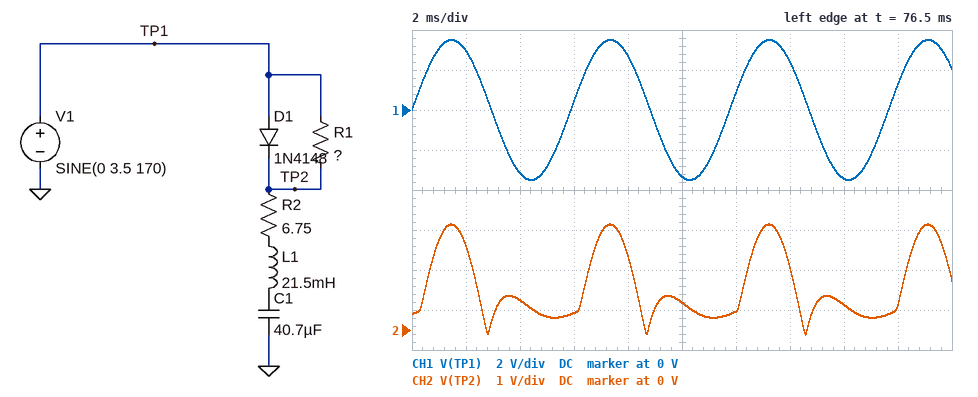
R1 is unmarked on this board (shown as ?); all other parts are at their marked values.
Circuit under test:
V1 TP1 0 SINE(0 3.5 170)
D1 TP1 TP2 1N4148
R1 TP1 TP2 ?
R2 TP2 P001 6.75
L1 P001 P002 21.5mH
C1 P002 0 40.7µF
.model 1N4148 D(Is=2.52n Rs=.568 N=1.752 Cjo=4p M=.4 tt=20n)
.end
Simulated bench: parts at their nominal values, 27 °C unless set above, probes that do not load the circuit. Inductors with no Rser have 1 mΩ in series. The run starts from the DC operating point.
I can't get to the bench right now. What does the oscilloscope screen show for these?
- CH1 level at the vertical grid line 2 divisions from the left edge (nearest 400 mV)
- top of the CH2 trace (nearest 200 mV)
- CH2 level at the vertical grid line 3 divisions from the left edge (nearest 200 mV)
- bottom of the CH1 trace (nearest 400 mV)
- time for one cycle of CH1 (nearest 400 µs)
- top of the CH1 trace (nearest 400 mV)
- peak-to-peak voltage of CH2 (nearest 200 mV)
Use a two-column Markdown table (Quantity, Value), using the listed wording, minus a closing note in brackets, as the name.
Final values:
| Quantity | Value |
|---|---|
| CH1 level at the vertical grid line 2 divisions from the left edge | -3.2 V |
| top of the CH2 trace | 2.6 V |
| CH2 level at the vertical grid line 3 divisions from the left edge | 400 mV |
| bottom of the CH1 trace | -3.6 V |
| time for one cycle of CH1 | 6.0 ms |
| top of the CH1 trace | 3.6 V |
| peak-to-peak voltage of CH2 | 2.8 V |
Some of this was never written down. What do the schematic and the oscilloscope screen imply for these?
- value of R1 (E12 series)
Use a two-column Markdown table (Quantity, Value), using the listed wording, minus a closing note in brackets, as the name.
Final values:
| Quantity | Value |
|---|---|
| value of R1 | 33 Ω |
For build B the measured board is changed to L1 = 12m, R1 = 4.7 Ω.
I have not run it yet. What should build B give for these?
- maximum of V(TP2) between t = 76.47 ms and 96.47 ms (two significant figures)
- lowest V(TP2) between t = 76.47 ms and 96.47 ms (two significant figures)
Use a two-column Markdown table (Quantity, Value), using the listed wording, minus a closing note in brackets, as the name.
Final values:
| Quantity | Value |
|---|---|
| maximum of V(TP2) between t = 76.47 ms and 96.47 ms | 2.8 V |
| lowest V(TP2) between t = 76.47 ms and 96.47 ms | -2.8 V |
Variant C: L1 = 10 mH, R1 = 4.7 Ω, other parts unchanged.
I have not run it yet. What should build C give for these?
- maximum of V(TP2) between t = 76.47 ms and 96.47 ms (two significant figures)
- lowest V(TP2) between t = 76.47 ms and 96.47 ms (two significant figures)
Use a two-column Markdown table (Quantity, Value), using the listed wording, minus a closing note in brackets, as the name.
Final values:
| Quantity | Value |
|---|---|
| maximum of V(TP2) between t = 76.47 ms and 96.47 ms | 2.9 V |
| lowest V(TP2) between t = 76.47 ms and 96.47 ms | -2.9 V |
